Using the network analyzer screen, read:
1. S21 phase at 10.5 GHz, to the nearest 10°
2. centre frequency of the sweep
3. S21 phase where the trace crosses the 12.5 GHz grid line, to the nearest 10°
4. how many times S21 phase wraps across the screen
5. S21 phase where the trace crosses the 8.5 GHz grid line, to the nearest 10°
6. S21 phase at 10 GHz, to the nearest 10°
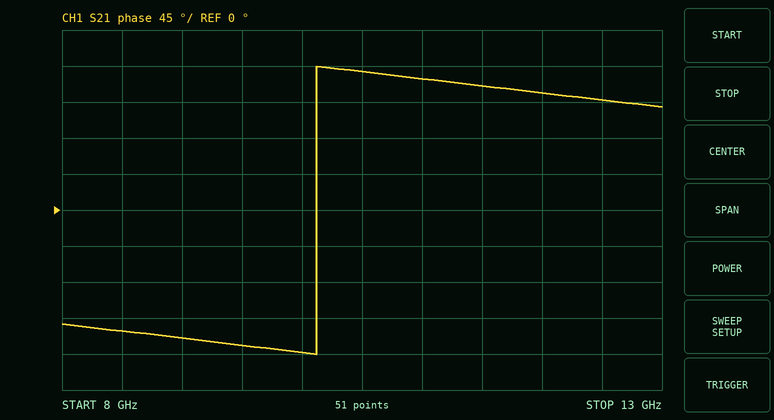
170°
10.5 GHz
140°
1
-150°
-180°
